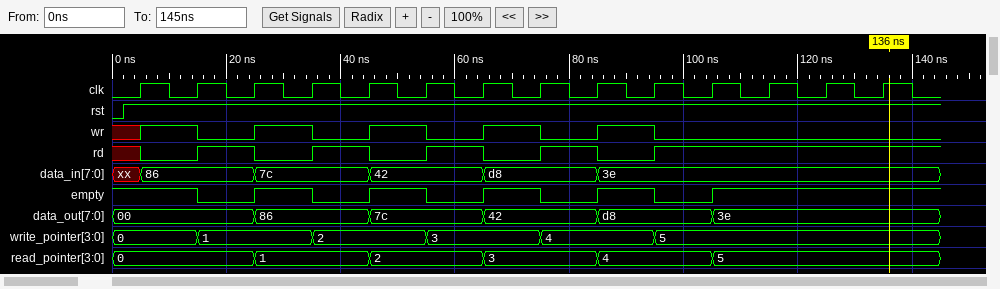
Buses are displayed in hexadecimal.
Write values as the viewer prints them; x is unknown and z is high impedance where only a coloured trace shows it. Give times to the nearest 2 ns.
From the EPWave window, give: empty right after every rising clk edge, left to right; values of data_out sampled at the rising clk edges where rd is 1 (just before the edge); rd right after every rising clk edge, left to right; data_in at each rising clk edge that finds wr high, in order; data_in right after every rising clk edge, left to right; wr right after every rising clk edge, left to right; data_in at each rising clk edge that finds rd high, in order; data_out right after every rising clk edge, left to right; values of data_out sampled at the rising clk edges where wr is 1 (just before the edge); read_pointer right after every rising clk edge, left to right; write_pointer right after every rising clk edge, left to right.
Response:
1 0 1 0 1 0 1 0 1 0 1 1 1 1
00, 86, 7c, 42, d8, 3e, 3e, 3e
0 1 0 1 0 1 0 1 0 1 1 1 1 1
86, 7c, 42, d8, 3e
86, 86, 7c, 7c, 42, 42, d8, d8, 3e, 3e, 3e, 3e, 3e, 3e
1 0 1 0 1 0 1 0 1 0 0 0 0 0
86, 7c, 42, d8, 3e, 3e, 3e, 3e
00, 00, 86, 86, 7c, 7c, 42, 42, d8, d8, 3e, 3e, 3e, 3e
00, 86, 7c, 42, d8
0, 0, 1, 1, 2, 2, 3, 3, 4, 4, 5, 5, 5, 5
0, 1, 1, 2, 2, 3, 3, 4, 4, 5, 5, 5, 5, 5
